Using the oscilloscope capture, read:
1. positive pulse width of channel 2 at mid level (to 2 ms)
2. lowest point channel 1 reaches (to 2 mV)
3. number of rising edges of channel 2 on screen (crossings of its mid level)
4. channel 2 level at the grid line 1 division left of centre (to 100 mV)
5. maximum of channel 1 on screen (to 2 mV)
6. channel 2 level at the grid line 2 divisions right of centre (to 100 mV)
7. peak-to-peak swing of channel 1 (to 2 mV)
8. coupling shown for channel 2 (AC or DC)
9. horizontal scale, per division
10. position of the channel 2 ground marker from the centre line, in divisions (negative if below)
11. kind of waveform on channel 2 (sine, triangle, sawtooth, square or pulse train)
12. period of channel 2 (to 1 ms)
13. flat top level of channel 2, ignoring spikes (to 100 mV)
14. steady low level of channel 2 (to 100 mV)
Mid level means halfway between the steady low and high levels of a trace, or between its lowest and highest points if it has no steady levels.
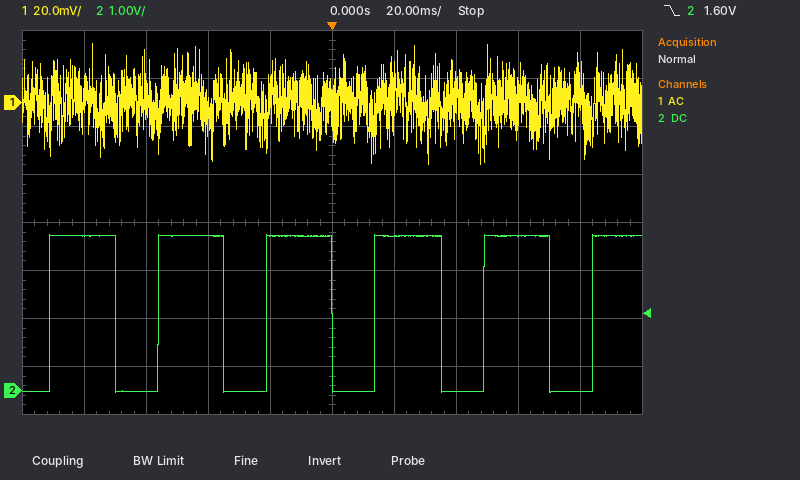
22 ms
-26 mV
6
3.2 V
24 mV
0.0 V
50 mV
DC
20 ms
-3.5 div
pulse train
35 ms
3.2 V
0.0 V
